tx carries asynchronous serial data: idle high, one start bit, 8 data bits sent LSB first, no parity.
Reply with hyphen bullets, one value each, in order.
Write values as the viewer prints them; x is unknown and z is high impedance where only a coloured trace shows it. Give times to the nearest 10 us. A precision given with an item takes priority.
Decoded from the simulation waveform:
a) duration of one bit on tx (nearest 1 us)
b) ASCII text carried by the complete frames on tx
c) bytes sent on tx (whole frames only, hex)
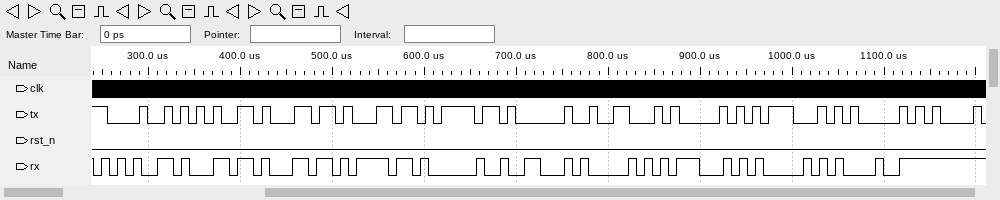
- 9 us
- "Hello FPGA"
- 48, 65, 6C, 6C, 6F, 20, 46, 50, 47, 41
